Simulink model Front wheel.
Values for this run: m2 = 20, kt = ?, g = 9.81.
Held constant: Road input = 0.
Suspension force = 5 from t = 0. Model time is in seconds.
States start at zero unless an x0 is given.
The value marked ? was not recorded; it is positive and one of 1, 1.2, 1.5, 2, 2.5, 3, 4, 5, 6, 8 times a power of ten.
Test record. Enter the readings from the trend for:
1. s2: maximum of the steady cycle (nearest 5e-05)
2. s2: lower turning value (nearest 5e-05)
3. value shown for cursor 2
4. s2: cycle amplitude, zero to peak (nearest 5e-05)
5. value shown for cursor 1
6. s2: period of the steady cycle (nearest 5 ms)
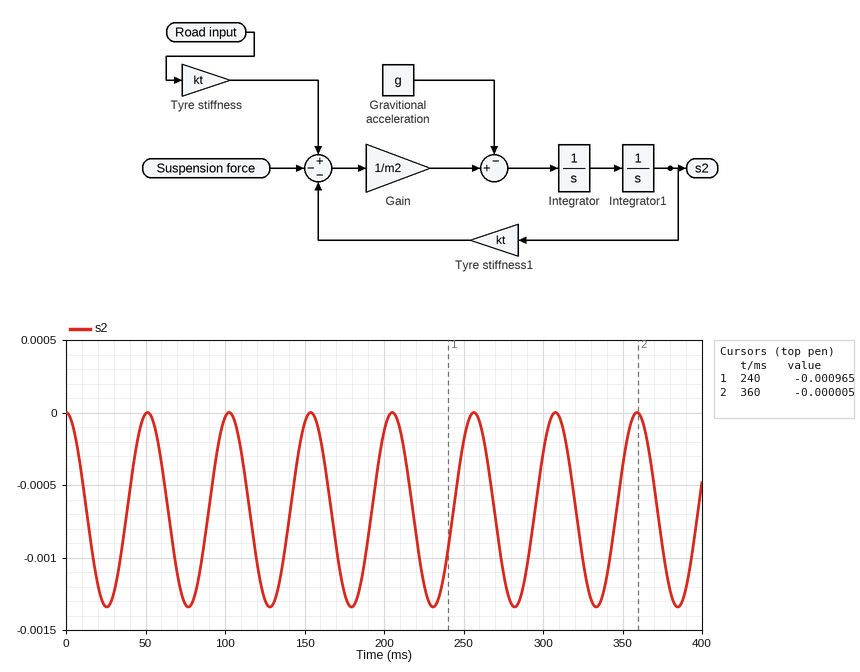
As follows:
0.00000
-0.00135
-0.000005
0.00065
-0.000965
50 ms
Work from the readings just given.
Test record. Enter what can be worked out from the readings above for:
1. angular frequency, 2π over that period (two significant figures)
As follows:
0.13 rad/ms
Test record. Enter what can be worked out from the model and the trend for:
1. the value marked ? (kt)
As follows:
300000
